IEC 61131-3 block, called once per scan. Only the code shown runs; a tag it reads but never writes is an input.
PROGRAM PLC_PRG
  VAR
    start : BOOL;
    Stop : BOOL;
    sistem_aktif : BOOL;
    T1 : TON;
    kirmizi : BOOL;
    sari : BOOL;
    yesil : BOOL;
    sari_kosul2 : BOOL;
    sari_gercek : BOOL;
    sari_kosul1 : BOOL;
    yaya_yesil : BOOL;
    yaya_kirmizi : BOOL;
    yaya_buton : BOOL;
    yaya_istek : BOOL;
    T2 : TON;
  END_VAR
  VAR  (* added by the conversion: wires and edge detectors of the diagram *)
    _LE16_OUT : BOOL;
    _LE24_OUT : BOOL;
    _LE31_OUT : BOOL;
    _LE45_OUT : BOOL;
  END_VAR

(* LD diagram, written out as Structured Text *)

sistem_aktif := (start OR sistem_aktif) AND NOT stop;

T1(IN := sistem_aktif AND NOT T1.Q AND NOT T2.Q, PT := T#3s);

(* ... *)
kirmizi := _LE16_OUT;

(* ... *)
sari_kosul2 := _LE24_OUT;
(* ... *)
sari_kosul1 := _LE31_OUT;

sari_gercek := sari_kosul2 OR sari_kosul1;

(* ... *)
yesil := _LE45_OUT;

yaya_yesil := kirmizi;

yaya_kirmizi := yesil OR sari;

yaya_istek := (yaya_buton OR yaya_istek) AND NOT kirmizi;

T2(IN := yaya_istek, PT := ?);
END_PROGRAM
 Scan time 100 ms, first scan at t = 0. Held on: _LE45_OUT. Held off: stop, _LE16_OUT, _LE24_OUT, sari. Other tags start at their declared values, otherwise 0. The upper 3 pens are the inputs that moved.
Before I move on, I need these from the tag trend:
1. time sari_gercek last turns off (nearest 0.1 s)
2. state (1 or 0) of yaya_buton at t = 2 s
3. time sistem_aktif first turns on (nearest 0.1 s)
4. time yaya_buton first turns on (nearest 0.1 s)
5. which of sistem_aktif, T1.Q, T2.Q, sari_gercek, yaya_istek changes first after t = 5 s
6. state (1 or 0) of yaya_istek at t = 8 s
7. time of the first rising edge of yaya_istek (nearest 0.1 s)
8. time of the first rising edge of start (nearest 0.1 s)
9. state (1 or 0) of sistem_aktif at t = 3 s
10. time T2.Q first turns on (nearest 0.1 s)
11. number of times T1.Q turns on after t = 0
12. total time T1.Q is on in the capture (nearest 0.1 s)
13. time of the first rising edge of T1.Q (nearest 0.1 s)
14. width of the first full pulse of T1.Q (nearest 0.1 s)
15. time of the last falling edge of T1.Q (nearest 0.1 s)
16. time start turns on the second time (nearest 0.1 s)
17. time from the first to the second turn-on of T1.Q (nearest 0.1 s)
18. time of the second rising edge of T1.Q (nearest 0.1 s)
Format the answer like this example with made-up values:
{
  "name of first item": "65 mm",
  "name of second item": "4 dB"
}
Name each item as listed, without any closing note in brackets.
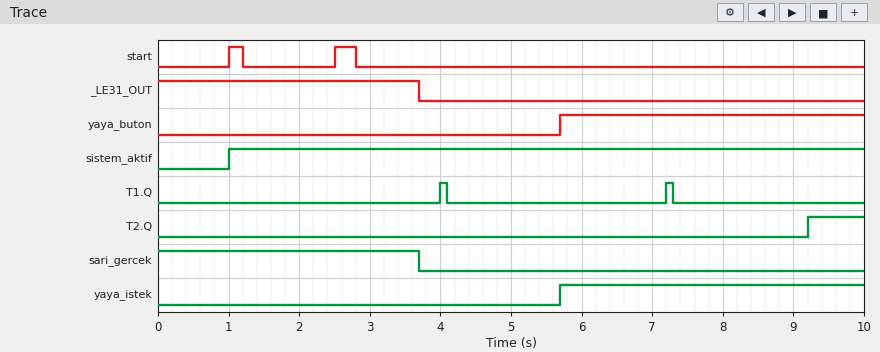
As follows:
{
  "time sari_gercek last turns off": "3.7 s",
  "state (1 or 0) of yaya_buton at t = 2 s": "0",
  "time sistem_aktif first turns on": "1.0 s",
  "time yaya_buton first turns on": "5.7 s",
  "which of sistem_aktif, T1.Q, T2.Q, sari_gercek, yaya_istek changes first after t = 5 s": "yaya_istek",
  "state (1 or 0) of yaya_istek at t = 8 s": "1",
  "time of the first rising edge of yaya_istek": "5.7 s",
  "time of the first rising edge of start": "1.0 s",
  "state (1 or 0) of sistem_aktif at t = 3 s": "1",
  "time T2.Q first turns on": "9.2 s",
  "number of times T1.Q turns on after t = 0": "2",
  "total time T1.Q is on in the capture": "0.2 s",
  "time of the first rising edge of T1.Q": "4.0 s",
  "width of the first full pulse of T1.Q": "0.1 s",
  "time of the last falling edge of T1.Q": "7.3 s",
  "time start turns on the second time": "2.5 s",
  "time from the first to the second turn-on of T1.Q": "3.2 s",
  "time of the second rising edge of T1.Q": "7.2 s"
}
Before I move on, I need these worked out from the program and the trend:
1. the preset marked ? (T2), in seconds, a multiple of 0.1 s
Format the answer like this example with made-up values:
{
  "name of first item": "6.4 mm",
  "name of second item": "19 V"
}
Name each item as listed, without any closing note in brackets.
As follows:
{
  "the preset marked ? (T2), in seconds, a multiple of 0.1 s": "3.5 s"
}
